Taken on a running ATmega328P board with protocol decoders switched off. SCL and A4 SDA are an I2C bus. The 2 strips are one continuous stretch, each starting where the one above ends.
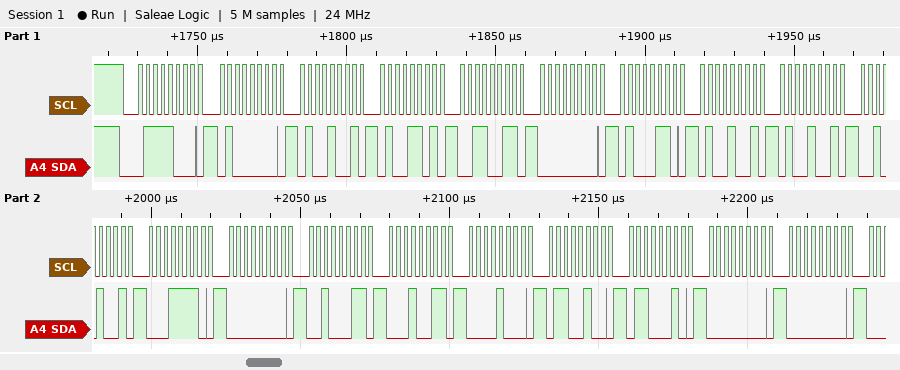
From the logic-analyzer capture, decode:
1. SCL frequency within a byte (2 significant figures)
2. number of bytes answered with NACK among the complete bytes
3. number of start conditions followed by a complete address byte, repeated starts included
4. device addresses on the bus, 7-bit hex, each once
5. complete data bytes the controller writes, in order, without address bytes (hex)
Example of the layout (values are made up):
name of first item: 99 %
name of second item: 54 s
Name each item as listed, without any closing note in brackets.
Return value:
SCL frequency within a byte: 400 kHz
number of bytes answered with NACK among the complete bytes: 0
number of start conditions followed by a complete address byte, repeated starts included: 1
device addresses on the bus, 7-bit hex, each once: 0x3C
complete data bytes the controller writes, in order, without address bytes: 40 49 4D 33 00 46 49 49 29 1E 00 23 13 08 64 62 00 00
